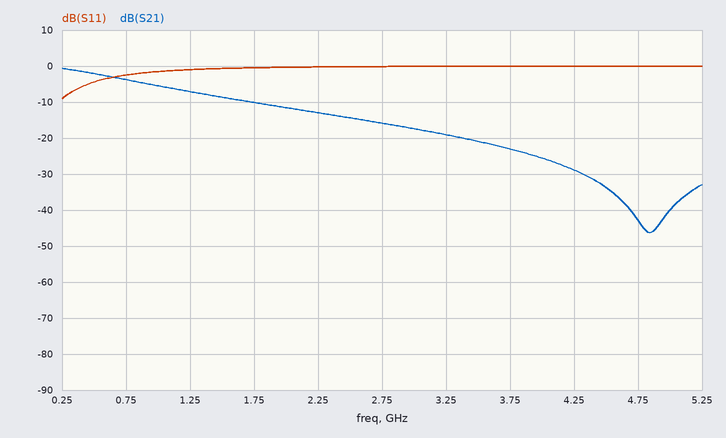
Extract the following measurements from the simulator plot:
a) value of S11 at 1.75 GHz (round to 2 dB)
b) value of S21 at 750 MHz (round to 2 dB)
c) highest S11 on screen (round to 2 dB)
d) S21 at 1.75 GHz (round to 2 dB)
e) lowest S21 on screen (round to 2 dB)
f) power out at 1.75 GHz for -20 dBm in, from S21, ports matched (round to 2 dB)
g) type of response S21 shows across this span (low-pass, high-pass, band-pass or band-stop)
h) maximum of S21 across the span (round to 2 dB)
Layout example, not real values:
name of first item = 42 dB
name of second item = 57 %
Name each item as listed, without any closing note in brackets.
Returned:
value of S11 at 1.75 GHz = 0 dB
value of S21 at 750 MHz = -4 dB
highest S11 on screen = 0 dB
S21 at 1.75 GHz = -10 dB
lowest S21 on screen = -46 dB
power out at 1.75 GHz for -20 dBm in, from S21, ports matched = -30 dBm
type of response S21 shows across this span = low-pass
maximum of S21 across the span = 0 dB
